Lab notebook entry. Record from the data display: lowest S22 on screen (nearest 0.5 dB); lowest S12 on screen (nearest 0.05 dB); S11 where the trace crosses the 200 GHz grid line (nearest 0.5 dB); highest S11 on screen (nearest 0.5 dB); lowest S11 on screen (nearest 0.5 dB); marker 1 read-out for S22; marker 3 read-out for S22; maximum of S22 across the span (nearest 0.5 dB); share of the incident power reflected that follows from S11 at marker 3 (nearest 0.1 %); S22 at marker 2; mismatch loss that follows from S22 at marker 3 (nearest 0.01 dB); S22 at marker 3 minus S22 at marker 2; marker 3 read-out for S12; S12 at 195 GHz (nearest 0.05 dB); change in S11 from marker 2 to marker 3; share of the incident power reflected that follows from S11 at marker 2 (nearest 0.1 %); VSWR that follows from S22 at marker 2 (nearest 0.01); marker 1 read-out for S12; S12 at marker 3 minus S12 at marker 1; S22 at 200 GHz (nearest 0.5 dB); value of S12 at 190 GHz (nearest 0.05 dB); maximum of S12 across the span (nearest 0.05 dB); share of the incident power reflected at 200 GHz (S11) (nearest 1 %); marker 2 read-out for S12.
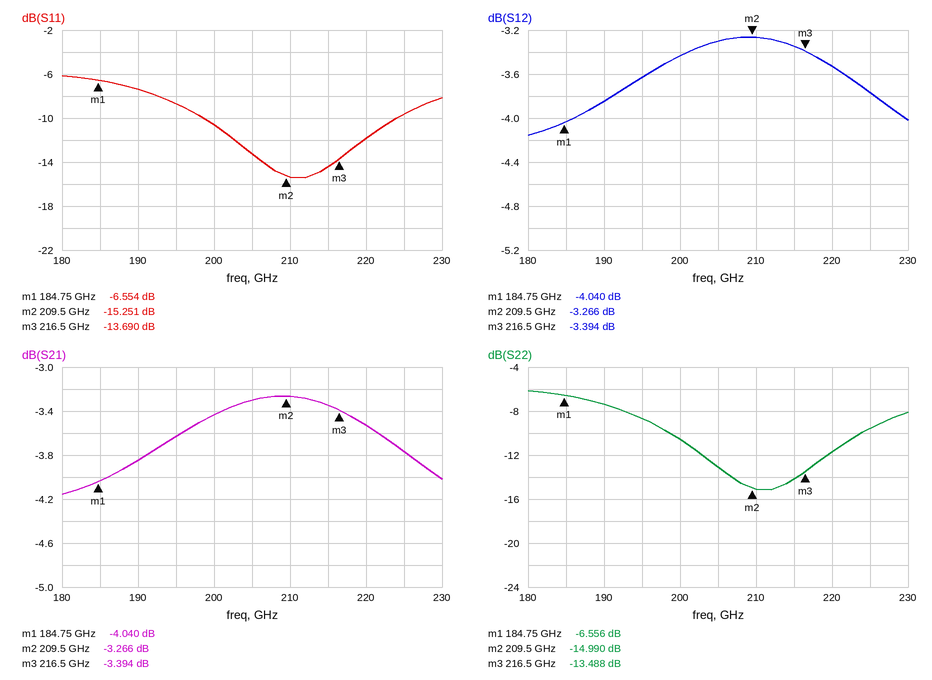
-15.0 dB
-4.15 dB
-10.5 dB
-6.0 dB
-15.5 dB
-6.556 dB
-13.488 dB
-6.0 dB
4.3 %
-14.990 dB
0.20 dB
1.502 dB
-3.394 dB
-3.65 dB
1.561 dB
3.0 %
1.43
-4.040 dB
0.646 dB
-10.5 dB
-3.85 dB
-3.25 dB
9 %
-3.266 dB
